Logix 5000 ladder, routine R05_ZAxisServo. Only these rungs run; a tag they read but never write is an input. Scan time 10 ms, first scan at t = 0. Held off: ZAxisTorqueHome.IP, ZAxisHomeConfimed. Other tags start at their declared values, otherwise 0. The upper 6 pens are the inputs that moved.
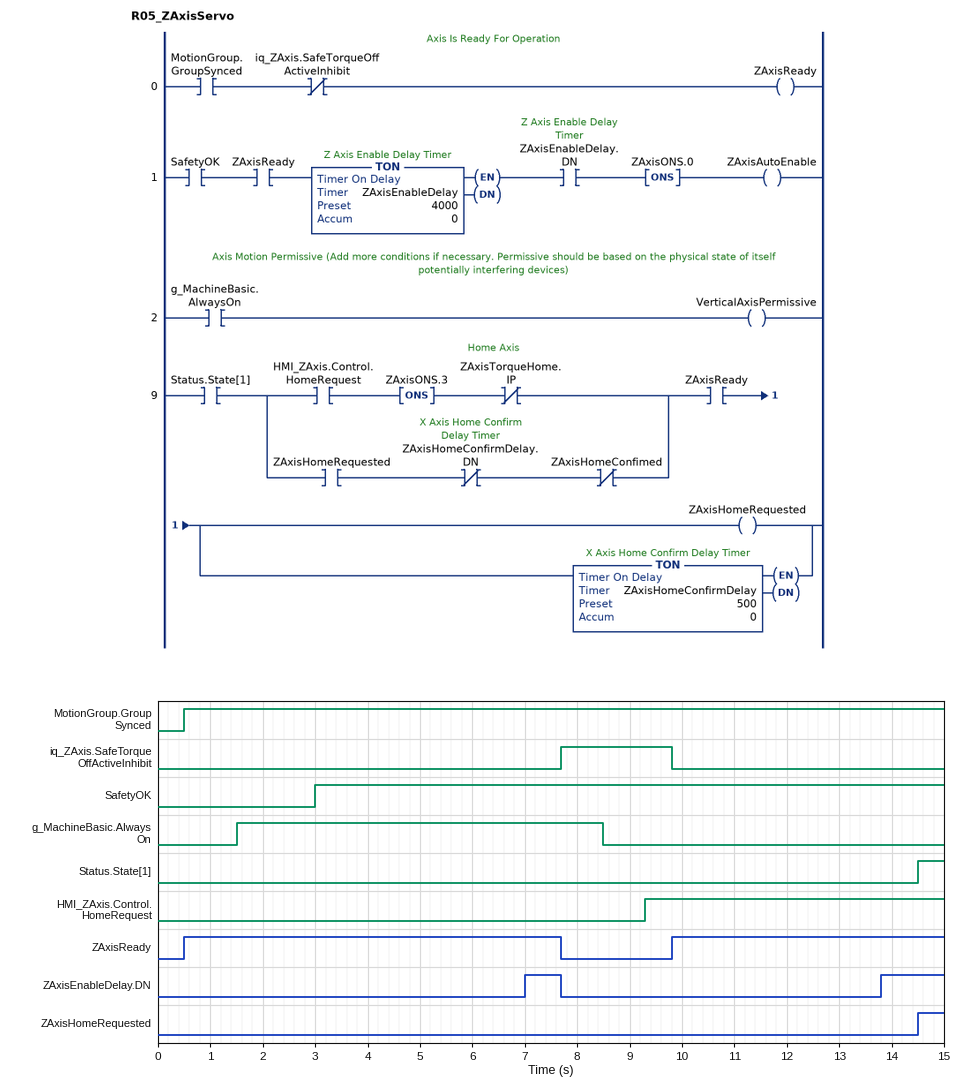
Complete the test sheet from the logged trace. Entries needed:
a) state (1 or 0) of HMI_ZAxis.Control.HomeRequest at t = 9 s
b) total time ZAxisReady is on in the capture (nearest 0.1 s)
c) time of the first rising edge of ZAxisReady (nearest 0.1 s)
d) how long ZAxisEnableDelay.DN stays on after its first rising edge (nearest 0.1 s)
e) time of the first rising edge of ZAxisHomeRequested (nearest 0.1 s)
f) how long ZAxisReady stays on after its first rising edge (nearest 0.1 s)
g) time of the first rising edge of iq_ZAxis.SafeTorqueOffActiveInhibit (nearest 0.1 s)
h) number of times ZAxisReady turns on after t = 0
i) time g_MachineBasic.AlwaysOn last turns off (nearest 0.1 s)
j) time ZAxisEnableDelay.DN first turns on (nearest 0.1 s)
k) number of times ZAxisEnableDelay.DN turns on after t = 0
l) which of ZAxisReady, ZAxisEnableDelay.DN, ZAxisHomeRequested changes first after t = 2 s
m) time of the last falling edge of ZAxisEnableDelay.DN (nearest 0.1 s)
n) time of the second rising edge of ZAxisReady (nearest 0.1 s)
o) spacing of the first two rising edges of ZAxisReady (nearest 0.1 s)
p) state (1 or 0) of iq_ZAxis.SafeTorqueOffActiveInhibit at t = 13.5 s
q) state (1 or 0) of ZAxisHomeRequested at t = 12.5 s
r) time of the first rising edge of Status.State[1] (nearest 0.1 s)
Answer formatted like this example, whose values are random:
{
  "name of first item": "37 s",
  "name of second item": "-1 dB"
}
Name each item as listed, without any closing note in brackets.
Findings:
{
  "state (1 or 0) of HMI_ZAxis.Control.HomeRequest at t = 9 s": "0",
  "total time ZAxisReady is on in the capture": "12.4 s",
  "time of the first rising edge of ZAxisReady": "0.5 s",
  "how long ZAxisEnableDelay.DN stays on after its first rising edge": "0.7 s",
  "time of the first rising edge of ZAxisHomeRequested": "14.5 s",
  "how long ZAxisReady stays on after its first rising edge": "7.2 s",
  "time of the first rising edge of iq_ZAxis.SafeTorqueOffActiveInhibit": "7.7 s",
  "number of times ZAxisReady turns on after t = 0": "2",
  "time g_MachineBasic.AlwaysOn last turns off": "8.5 s",
  "time ZAxisEnableDelay.DN first turns on": "7.0 s",
  "number of times ZAxisEnableDelay.DN turns on after t = 0": "2",
  "which of ZAxisReady, ZAxisEnableDelay.DN, ZAxisHomeRequested changes first after t = 2 s": "ZAxisEnableDelay.DN",
  "time of the last falling edge of ZAxisEnableDelay.DN": "7.7 s",
  "time of the second rising edge of ZAxisReady": "9.8 s",
  "spacing of the first two rising edges of ZAxisReady": "9.3 s",
  "state (1 or 0) of iq_ZAxis.SafeTorqueOffActiveInhibit at t = 13.5 s": "0",
  "state (1 or 0) of ZAxisHomeRequested at t = 12.5 s": "0",
  "time of the first rising edge of Status.State[1]": "14.5 s"
}
